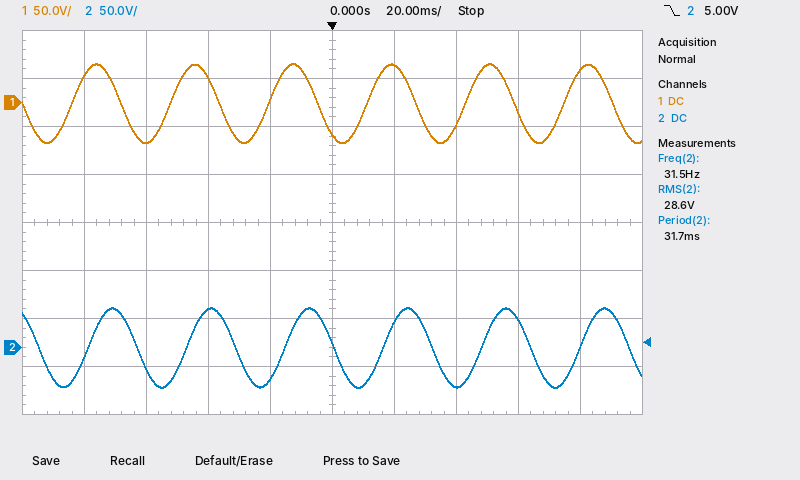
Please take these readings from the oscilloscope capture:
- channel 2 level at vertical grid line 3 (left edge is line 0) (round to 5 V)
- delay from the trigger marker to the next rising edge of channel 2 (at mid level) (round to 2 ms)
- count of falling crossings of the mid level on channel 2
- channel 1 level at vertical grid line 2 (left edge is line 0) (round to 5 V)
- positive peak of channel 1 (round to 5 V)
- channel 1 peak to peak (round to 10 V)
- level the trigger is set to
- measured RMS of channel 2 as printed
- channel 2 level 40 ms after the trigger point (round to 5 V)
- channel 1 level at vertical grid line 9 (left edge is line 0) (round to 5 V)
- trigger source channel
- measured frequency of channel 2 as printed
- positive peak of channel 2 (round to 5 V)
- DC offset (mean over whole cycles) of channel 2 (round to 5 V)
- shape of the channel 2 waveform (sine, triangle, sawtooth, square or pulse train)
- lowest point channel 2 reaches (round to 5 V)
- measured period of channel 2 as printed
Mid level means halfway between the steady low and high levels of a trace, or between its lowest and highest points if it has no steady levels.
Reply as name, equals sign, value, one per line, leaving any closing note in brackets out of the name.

channel 2 level at vertical grid line 3 (left edge is line 0) = 40 V
delay from the trigger marker to the next rising edge of channel 2 (at mid level) = 16 ms
count of falling crossings of the mid level on channel 2 = 7
channel 1 level at vertical grid line 2 (left edge is line 0) = -40 V
positive peak of channel 1 = 40 V
channel 1 peak to peak = 80 V
level the trigger is set to = 5.00 V
measured RMS of channel 2 as printed = 28.6 V
channel 2 level 40 ms after the trigger point = -40 V
channel 1 level at vertical grid line 9 (left edge is line 0) = 35 V
trigger source channel = channel 2
measured frequency of channel 2 as printed = 31.5 Hz
positive peak of channel 2 = 40 V
DC offset (mean over whole cycles) of channel 2 = 0 V
shape of the channel 2 waveform = sine
lowest point channel 2 reaches = -40 V
measured period of channel 2 as printed = 31.7 ms
